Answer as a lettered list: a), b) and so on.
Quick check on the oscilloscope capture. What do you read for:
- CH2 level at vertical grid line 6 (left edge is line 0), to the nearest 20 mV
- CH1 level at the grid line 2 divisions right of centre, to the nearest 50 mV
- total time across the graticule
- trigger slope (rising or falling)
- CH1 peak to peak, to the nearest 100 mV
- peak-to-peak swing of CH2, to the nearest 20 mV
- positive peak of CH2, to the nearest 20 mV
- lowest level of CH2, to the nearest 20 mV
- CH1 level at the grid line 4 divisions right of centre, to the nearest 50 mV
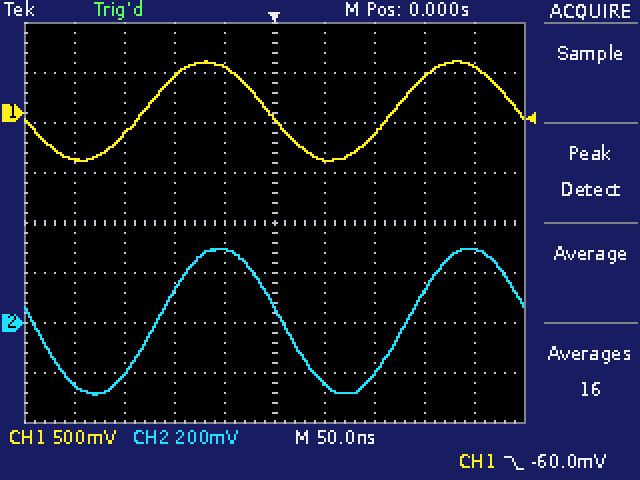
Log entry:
a) -240 mV
b) -200 mV
c) 500 ns
d) falling
e) 1.00 V
f) 580 mV
g) 300 mV
h) -280 mV
i) 450 mV
